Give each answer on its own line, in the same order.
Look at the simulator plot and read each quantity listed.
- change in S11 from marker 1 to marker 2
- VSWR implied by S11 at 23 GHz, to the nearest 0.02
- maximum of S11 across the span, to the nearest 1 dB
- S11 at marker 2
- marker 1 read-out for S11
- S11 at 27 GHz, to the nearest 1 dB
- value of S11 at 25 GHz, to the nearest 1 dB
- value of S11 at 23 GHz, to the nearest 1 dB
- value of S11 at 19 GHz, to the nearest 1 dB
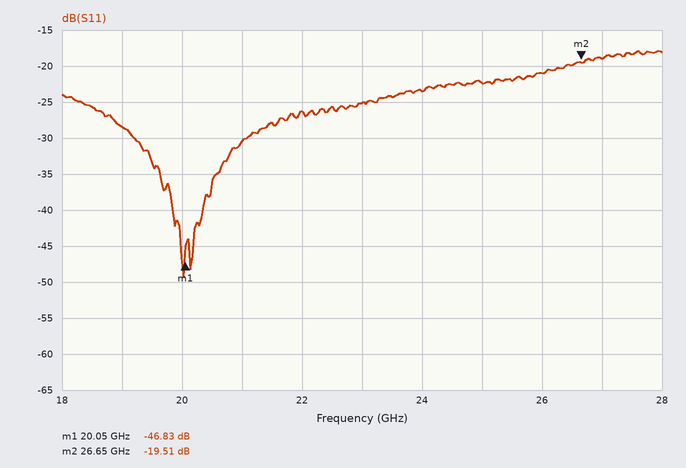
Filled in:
27.32 dB
1.12
-18 dB
-19.51 dB
-46.83 dB
-19 dB
-22 dB
-25 dB
-28 dB
